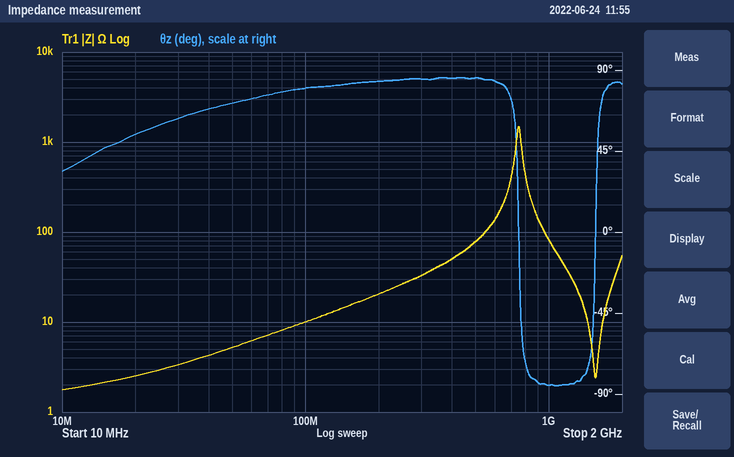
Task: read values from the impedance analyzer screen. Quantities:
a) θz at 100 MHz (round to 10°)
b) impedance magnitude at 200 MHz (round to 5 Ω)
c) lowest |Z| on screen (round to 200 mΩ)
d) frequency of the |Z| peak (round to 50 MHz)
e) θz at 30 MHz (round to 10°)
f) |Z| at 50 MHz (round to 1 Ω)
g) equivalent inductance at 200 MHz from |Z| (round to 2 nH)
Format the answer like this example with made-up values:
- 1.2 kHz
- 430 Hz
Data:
- 80°
- 20 Ω
- 1.8 Ω
- 750 MHz
- 60°
- 5 Ω
- 16 nH
